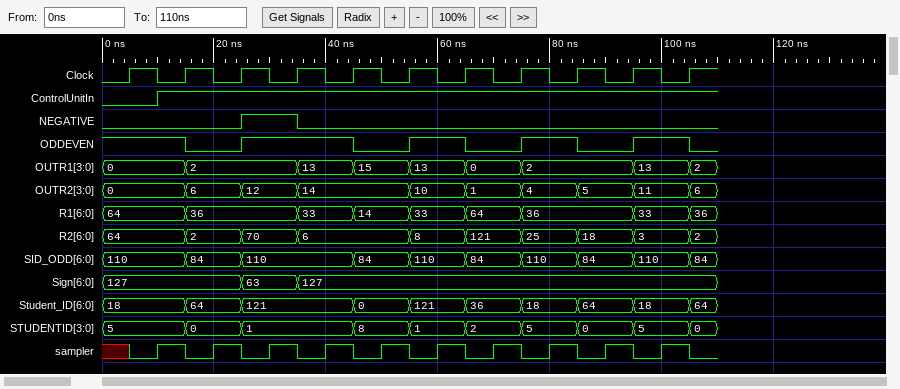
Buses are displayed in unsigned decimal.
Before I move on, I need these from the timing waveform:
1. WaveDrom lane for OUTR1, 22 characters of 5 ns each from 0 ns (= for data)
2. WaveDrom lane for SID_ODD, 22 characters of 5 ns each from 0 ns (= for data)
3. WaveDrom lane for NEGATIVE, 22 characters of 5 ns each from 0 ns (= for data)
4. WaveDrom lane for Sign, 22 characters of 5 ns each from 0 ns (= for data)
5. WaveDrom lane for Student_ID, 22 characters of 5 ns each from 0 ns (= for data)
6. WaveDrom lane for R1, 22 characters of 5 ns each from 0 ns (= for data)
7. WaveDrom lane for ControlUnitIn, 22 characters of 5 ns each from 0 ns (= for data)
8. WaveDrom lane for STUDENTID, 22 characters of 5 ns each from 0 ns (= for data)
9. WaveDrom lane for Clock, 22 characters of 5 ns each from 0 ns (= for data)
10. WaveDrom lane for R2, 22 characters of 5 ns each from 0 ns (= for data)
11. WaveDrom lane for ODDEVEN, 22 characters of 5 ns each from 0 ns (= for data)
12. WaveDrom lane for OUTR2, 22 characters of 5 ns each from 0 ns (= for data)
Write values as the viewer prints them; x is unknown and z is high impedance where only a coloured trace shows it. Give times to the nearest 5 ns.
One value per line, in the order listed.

{name: 'OUTR1', wave: '=..=...=.=.=.=.=...=.=', data: '0 2 13 15 13 0 2 13 2'}
{name: 'SID_ODD', wave: '=..=.=...=.=.=.=.=.=.=', data: '110 84 110 84 110 84 110 84 110 84'}
{name: 'NEGATIVE', wave: '0....1.0..............'}
{name: 'Sign', wave: '=....=.=..............', data: '127 63 127'}
{name: 'Student_ID', wave: '=..=.=...=.=.=.=.=.=.=', data: '18 64 121 0 121 36 18 64 18 64'}
{name: 'R1', wave: '=..=...=.=.=.=.=...=.=', data: '64 36 33 14 33 64 36 33 36'}
{name: 'ControlUnitIn', wave: '0.1...................'}
{name: 'STUDENTID', wave: '=..=.=...=.=.=.=.=.=.=', data: '5 0 1 8 1 2 5 0 5 0'}
{name: 'Clock', wave: '0101010101010101010101'}
{name: 'R2', wave: '=..=.=.=...=.=.=.=.=.=', data: '64 2 70 6 8 121 25 18 3 2'}
{name: 'ODDEVEN', wave: '1..0.1...0.1.0.1.0.1.0'}
{name: 'OUTR2', wave: '=..=.=.=...=.=.=.=.=.=', data: '0 6 12 14 10 1 4 5 11 6'}
